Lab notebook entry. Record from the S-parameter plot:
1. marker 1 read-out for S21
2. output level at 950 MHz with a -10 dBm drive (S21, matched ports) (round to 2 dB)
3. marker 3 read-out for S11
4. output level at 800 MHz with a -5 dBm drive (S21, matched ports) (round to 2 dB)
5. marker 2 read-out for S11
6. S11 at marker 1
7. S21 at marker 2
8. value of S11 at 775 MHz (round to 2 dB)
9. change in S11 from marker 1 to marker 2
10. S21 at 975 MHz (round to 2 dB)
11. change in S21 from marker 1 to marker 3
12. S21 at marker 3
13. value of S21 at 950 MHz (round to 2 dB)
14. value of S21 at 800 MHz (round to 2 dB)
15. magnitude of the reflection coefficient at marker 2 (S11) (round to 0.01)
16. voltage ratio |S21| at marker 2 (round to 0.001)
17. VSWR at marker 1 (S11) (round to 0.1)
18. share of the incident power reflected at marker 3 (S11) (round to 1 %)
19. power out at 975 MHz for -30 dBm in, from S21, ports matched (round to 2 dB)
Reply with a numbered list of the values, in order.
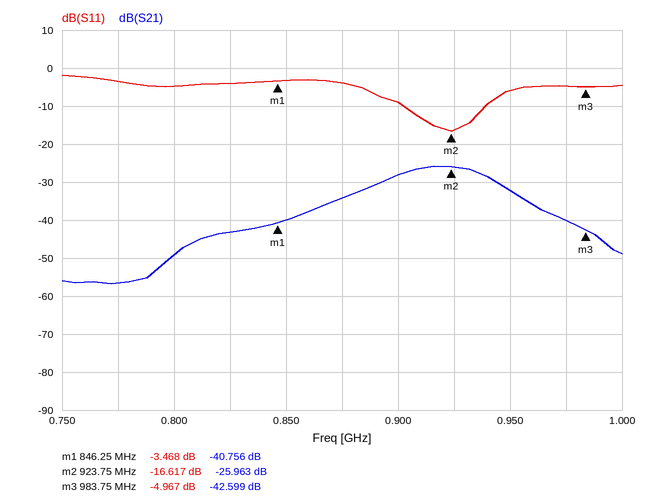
1. -40.756 dB
2. -42 dBm
3. -4.967 dB
4. -54 dBm
5. -16.617 dB
6. -3.468 dB
7. -25.963 dB
8. -4 dB
9. -13.149 dB
10. -40 dB
11. -1.843 dB
12. -42.599 dB
13. -32 dB
14. -50 dB
15. 0.15
16. 0.050
17. 5.1
18. 32 %
19. -70 dBm
